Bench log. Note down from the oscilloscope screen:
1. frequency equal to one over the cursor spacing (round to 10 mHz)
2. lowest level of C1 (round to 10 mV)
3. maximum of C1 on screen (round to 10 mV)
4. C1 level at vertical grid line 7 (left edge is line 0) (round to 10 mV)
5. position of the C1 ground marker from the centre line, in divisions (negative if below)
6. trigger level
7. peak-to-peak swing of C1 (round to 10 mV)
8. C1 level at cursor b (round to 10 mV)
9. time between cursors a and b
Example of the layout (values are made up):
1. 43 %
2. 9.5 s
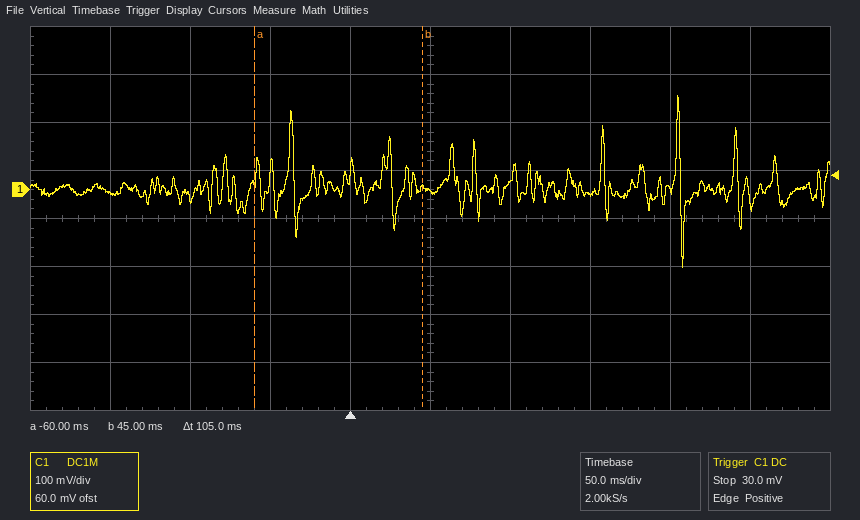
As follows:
1. 9.52 Hz
2. -160 mV
3. 200 mV
4. -10 mV
5. +0.6 div
6. 30.0 mV
7. 360 mV
8. 0 mV
9. 105 ms
